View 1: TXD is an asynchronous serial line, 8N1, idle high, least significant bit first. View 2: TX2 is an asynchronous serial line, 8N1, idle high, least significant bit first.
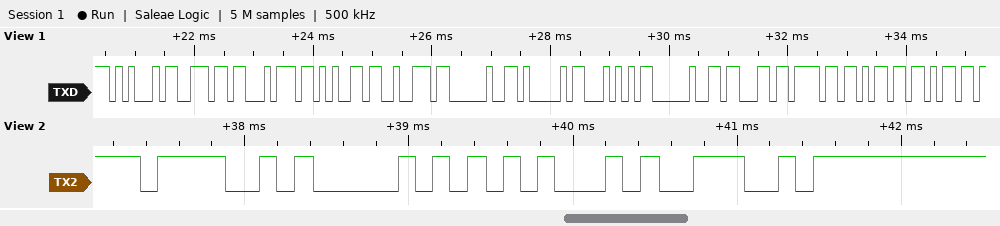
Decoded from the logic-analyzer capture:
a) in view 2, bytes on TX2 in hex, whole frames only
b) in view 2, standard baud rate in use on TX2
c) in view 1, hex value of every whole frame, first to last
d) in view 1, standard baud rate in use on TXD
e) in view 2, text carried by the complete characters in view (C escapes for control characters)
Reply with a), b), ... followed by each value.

a) 4F 50 45 4E
b) 9600 baud
c) 0x45 0x6E 0x74 0x65 0x72 0x20 0x41 0x54 0x20 0x63 0x6F 0x6D 0x6D
d) 9600 baud
e) "OPEN"
